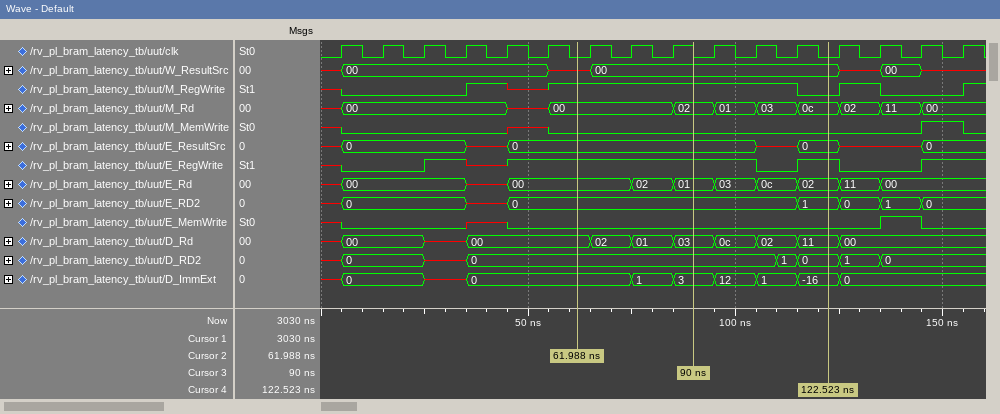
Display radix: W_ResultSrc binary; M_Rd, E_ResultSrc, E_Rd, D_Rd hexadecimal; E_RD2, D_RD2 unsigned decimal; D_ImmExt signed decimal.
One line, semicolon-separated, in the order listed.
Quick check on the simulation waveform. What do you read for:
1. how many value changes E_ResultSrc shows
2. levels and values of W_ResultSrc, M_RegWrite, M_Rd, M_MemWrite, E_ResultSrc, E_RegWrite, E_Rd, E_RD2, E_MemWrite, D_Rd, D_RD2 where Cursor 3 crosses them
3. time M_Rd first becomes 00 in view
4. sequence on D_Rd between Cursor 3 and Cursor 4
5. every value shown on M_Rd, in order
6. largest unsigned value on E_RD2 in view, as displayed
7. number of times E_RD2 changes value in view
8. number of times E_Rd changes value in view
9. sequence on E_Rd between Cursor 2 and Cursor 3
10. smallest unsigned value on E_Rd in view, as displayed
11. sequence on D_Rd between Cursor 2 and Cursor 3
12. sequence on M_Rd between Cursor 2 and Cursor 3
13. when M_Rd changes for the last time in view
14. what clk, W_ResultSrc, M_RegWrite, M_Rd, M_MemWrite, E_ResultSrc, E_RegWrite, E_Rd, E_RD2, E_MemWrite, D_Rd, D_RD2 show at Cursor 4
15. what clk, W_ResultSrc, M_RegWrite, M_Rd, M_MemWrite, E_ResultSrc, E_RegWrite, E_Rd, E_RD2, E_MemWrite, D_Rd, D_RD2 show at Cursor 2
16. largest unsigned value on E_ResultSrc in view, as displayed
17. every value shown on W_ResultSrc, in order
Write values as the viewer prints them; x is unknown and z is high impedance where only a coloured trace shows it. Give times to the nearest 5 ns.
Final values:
7; W_ResultSrc=00, M_RegWrite=1, M_Rd=02, M_MemWrite=0, E_ResultSrc=0, E_RegWrite=1, E_Rd=01, E_RD2=0, E_MemWrite=0, D_Rd=03, D_RD2=0; 5 ns; 03, 0c, 02, 11; x, 00, x, 00, 02, 01, 03, 0c, 02, 11, 00; 1; 7; 10; 00, 02, 01; 00; 00, 02, 01, 03; 00, 02; 145 ns; clk=0, W_ResultSrc=00, M_RegWrite=0, M_Rd=0c, M_MemWrite=0, E_ResultSrc=0, E_RegWrite=1, E_Rd=02, E_RD2=1, E_MemWrite=0, D_Rd=11, D_RD2=0; clk=0, W_ResultSrc=x, M_RegWrite=1, M_Rd=00, M_MemWrite=0, E_ResultSrc=0, E_RegWrite=1, E_Rd=00, E_RD2=0, E_MemWrite=0, D_Rd=00, D_RD2=0; 0; x, 00, x, 00, x, 00, x
